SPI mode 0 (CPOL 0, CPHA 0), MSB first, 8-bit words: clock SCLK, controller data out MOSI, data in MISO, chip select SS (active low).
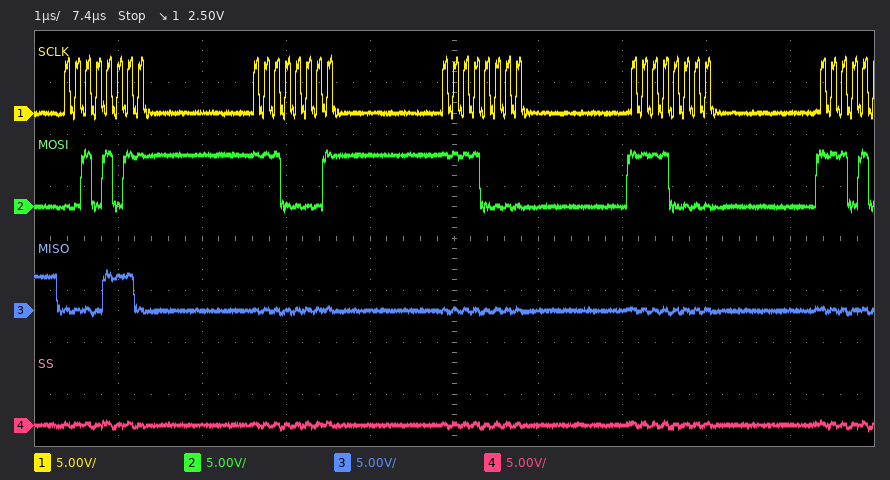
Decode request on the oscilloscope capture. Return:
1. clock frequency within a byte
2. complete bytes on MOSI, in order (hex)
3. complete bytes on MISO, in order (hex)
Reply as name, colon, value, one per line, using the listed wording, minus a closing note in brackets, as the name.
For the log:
clock frequency within a byte: 8 MHz
complete bytes on MOSI, in order: 0x2B 0xE1 0xF0 0xF0
complete bytes on MISO, in order: 0x0E 0x00 0x00 0x00
